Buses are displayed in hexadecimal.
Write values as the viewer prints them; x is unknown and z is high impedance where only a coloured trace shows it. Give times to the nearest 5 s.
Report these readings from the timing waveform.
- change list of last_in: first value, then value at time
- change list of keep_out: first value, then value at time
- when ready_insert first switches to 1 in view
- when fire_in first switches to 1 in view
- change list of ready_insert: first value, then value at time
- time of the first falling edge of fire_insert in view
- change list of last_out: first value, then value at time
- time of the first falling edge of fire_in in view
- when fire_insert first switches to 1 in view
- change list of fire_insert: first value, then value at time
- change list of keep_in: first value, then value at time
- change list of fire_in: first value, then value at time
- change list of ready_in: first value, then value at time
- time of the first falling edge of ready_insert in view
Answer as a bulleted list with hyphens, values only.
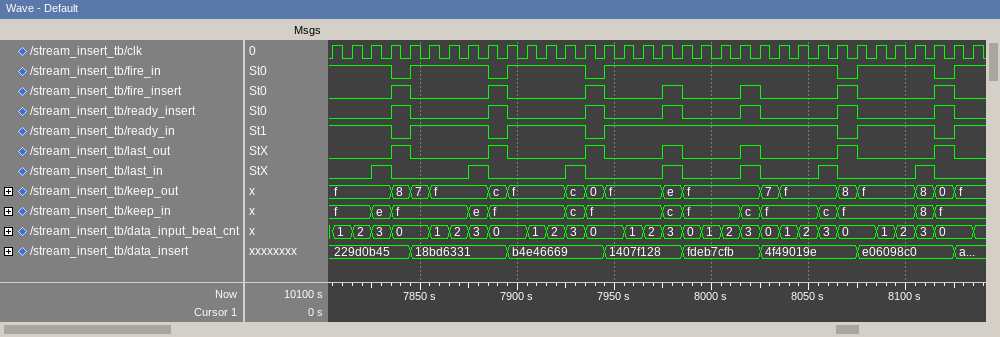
- 0, 1 at 7825 s, 0 at 7835 s, 1 at 7875 s, 0 at 7885 s, 1 at 7925 s, 0 at 7935 s, 1 at 7975 s, 0 at 7985 s, 1 at 8015 s, 0 at 8025 s, 1 at 8055 s, 0 at 8065 s, 1 at 8105 s, 0 at 8115 s
- f, 8 at 7835 s, 7 at 7845 s, f at 7855 s, c at 7885 s, f at 7895 s, c at 7925 s, 0 at 7935 s, f at 7945 s, e at 7975 s, f at 7985 s, 7 at 8025 s, f at 8035 s, 8 at 8065 s, f at 8075 s, 8 at 8105 s, 0 at 8115 s, f at 8125 s
- 7835 s
- 7845 s
- 0, 1 at 7835 s, 0 at 7845 s, 1 at 7885 s, 0 at 7895 s, 1 at 7935 s, 0 at 7945 s, 1 at 7975 s, 0 at 7985 s, 1 at 8015 s, 0 at 8025 s, 1 at 8065 s, 0 at 8075 s, 1 at 8115 s, 0 at 8125 s
- 7845 s
- 0, 1 at 7835 s, 0 at 7845 s, 1 at 7885 s, 0 at 7895 s, 1 at 7935 s, 0 at 7945 s, 1 at 7975 s, 0 at 7985 s, 1 at 8015 s, 0 at 8025 s, 1 at 8065 s, 0 at 8075 s, 1 at 8115 s, 0 at 8125 s
- 7835 s
- 7835 s
- 0, 1 at 7835 s, 0 at 7845 s, 1 at 7885 s, 0 at 7895 s, 1 at 7935 s, 0 at 7945 s, 1 at 7975 s, 0 at 7985 s, 1 at 8015 s, 0 at 8025 s, 1 at 8065 s, 0 at 8075 s, 1 at 8115 s, 0 at 8125 s
- f, e at 7825 s, f at 7835 s, e at 7875 s, f at 7885 s, c at 7925 s, f at 7935 s, c at 7975 s, f at 7985 s, c at 8015 s, f at 8025 s, c at 8055 s, f at 8065 s, 8 at 8105 s, f at 8115 s
- 1, 0 at 7835 s, 1 at 7845 s, 0 at 7885 s, 1 at 7895 s, 0 at 7935 s, 1 at 7945 s, 0 at 8065 s, 1 at 8075 s, 0 at 8115 s, 1 at 8125 s
- 1, 0 at 7835 s, 1 at 7845 s, 0 at 7885 s, 1 at 7895 s, 0 at 7935 s, 1 at 7945 s, 0 at 8065 s, 1 at 8075 s, 0 at 8115 s, 1 at 8125 s
- 7845 s
